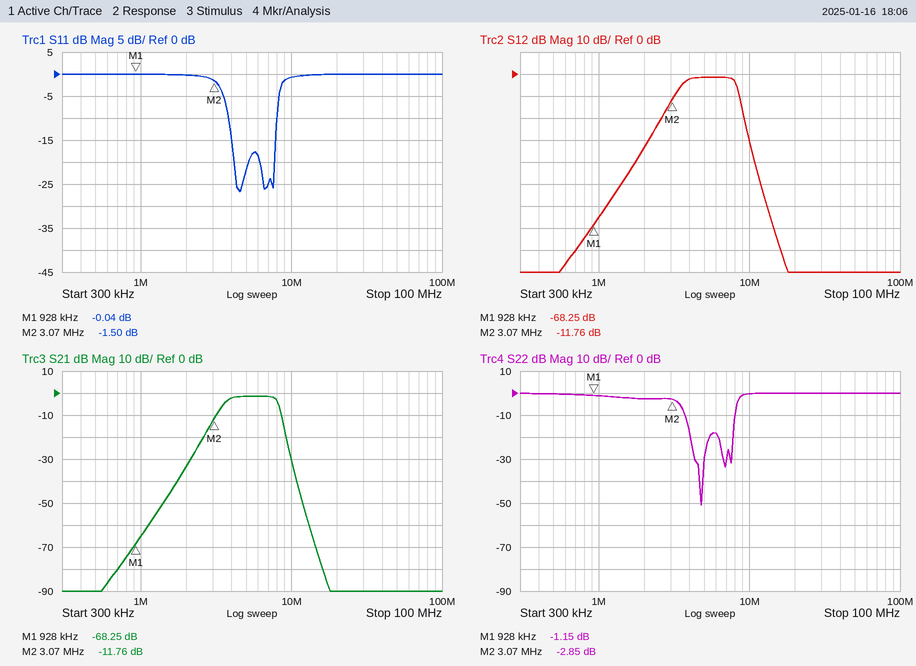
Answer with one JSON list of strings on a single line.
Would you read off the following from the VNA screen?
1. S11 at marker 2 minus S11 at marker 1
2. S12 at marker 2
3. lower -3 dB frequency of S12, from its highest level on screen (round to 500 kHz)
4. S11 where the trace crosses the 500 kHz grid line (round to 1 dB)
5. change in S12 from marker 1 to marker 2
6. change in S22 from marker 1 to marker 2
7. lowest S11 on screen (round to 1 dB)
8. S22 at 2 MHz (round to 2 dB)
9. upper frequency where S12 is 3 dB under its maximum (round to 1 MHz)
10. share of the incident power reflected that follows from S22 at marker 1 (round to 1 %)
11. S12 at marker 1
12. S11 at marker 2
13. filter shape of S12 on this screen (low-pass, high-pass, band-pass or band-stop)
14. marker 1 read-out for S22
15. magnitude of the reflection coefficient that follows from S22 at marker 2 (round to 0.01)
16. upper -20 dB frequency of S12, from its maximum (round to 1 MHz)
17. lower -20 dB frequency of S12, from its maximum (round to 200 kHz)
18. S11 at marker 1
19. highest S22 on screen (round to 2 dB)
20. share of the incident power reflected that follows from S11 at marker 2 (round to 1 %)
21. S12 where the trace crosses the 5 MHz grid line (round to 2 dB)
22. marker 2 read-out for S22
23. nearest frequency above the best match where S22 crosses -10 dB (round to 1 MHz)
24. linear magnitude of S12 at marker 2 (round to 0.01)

["-1.46 dB", "-11.76 dB", "3.5 MHz", "0 dB", "56.49 dB", "-1.70 dB", "-27 dB", "-2 dB", "8 MHz", "77 %", "-68.25 dB", "-1.50 dB", "band-pass", "-1.15 dB", "0.72", "9 MHz", "2.6 MHz", "-0.04 dB", "0 dB", "71 %", "-2 dB", "-2.85 dB", "8 MHz", "0.26"]
